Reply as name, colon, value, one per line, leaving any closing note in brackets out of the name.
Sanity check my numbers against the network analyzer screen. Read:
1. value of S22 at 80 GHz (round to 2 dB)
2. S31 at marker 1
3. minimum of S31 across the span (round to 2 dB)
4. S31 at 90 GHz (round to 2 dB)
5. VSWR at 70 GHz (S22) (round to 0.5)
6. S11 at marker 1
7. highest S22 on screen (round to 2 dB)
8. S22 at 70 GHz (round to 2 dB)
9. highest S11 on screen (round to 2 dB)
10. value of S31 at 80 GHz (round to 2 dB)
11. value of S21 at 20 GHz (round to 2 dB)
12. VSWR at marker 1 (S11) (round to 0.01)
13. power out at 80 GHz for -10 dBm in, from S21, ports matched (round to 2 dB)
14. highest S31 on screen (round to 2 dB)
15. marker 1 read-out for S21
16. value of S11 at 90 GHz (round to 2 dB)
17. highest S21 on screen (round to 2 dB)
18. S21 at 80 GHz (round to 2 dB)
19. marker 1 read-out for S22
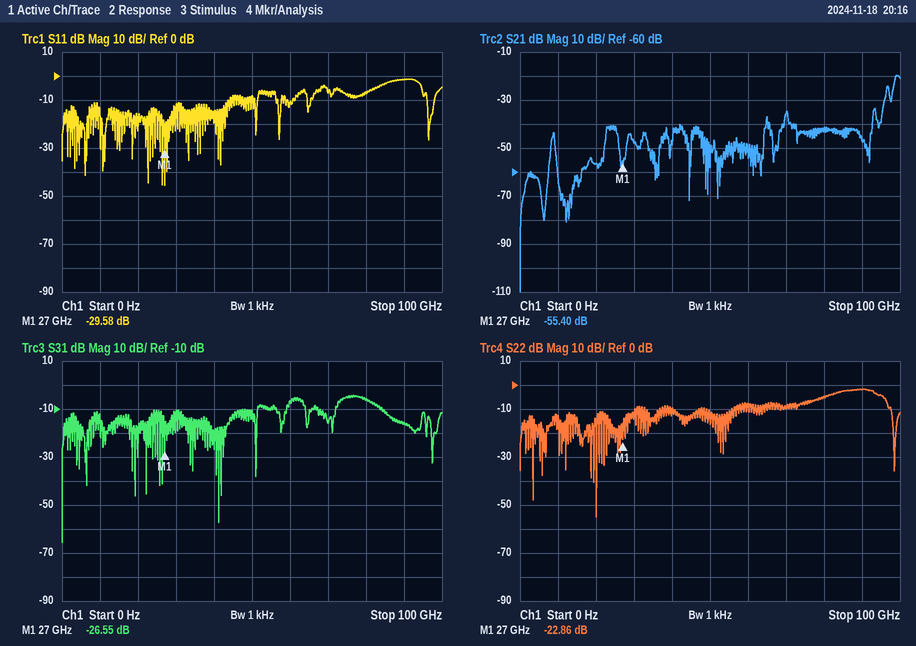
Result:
value of S22 at 80 GHz: -4 dB
S31 at marker 1: -26.55 dB
minimum of S31 across the span: -66 dB
S31 at 90 GHz: -16 dB
VSWR at 70 GHz (S22): 2.0
S11 at marker 1: -29.58 dB
highest S22 on screen: -2 dB
S22 at 70 GHz: -10 dB
highest S11 on screen: -2 dB
value of S31 at 80 GHz: -6 dB
value of S21 at 20 GHz: -56 dB
VSWR at marker 1 (S11): 1.07
power out at 80 GHz for -10 dBm in, from S21, ports matched: -52 dBm
highest S31 on screen: -4 dB
marker 1 read-out for S21: -55.40 dB
value of S11 at 90 GHz: -2 dB
highest S21 on screen: -20 dB
S21 at 80 GHz: -42 dB
marker 1 read-out for S22: -22.86 dB
